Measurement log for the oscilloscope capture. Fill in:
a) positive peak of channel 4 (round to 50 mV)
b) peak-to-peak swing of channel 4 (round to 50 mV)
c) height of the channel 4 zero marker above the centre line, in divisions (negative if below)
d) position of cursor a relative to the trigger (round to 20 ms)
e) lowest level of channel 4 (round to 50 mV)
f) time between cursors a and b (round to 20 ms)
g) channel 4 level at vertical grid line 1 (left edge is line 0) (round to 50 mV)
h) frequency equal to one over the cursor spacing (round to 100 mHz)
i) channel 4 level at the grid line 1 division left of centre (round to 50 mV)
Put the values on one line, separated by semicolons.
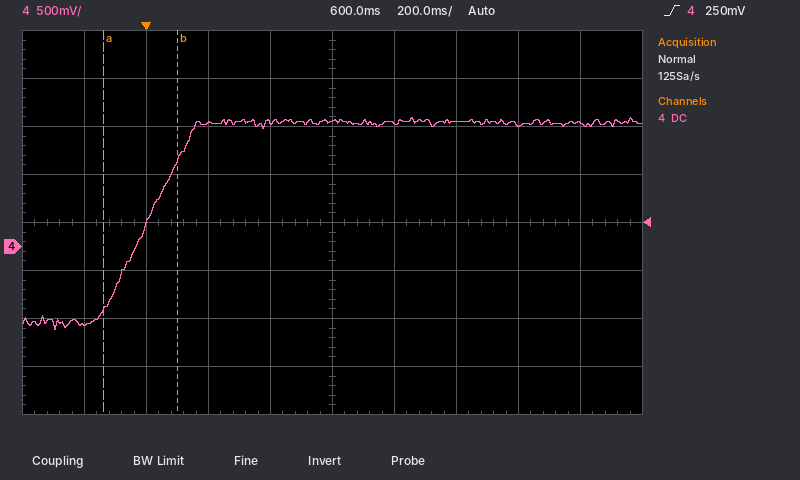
1.35 V; 2.20 V; -0.5 div; -140 ms; -850 mV; 240 ms; -800 mV; 4.2 Hz; 1.30 V
